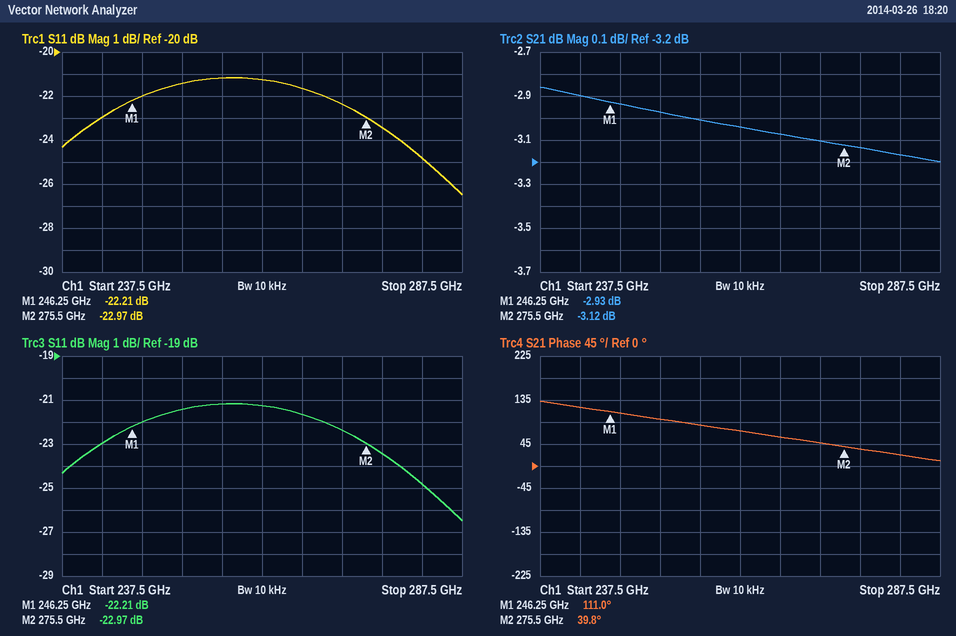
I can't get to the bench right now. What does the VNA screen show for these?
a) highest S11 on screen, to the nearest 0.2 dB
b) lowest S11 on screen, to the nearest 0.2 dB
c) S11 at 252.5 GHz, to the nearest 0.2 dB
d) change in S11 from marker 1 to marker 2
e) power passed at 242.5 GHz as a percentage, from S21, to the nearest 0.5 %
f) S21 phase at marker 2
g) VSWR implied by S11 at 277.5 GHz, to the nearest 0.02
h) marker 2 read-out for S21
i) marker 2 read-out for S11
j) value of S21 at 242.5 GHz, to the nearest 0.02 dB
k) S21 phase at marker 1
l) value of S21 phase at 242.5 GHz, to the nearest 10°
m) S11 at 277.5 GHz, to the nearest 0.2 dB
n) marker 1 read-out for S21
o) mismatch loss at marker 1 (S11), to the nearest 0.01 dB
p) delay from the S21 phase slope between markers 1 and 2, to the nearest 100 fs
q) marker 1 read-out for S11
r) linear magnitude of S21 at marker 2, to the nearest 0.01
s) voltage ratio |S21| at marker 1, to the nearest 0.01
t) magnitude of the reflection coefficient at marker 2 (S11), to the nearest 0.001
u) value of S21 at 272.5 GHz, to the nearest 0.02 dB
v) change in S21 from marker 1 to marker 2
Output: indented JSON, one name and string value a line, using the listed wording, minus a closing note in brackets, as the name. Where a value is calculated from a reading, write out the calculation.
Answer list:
{
  "highest S11 on screen, to the nearest 0.2 dB": "-21.2 dB",
  "lowest S11 on screen, to the nearest 0.2 dB": "-26.4 dB",
  "S11 at 252.5 GHz, to the nearest 0.2 dB": "-21.4 dB",
  "change in S11 from marker 1 to marker 2": "-22.97 − (-22.21) = -0.76 dB",
  "power passed at 242.5 GHz as a percentage, from S21, to the nearest 0.5 %": "10^(-2.9/10) ≈ 51.3 %, so 51.5 % to the nearest 0.5 %",
  "S21 phase at marker 2": "39.8°",
  "VSWR implied by S11 at 277.5 GHz, to the nearest 0.02": "|Γ| = 10^(-23.4/20) = 0.0676; VSWR = (1 + 0.0676)/(1 − 0.0676) ≈ 1.15, so 1.14 to the nearest 0.02",
  "marker 2 read-out for S21": "-3.12 dB",
  "marker 2 read-out for S11": "-22.97 dB",
  "value of S21 at 242.5 GHz, to the nearest 0.02 dB": "-2.90 dB",
  "S21 phase at marker 1": "111.0°",
  "value of S21 phase at 242.5 GHz, to the nearest 10°": "120°",
  "S11 at 277.5 GHz, to the nearest 0.2 dB": "-23.4 dB",
  "marker 1 read-out for S21": "-2.93 dB",
  "mismatch loss at marker 1 (S11), to the nearest 0.01 dB": "−10 log10(1 − 10^(-22.21/10)) ≈ 0.03 dB",
  "delay from the S21 phase slope between markers 1 and 2, to the nearest 100 fs": "−(39.8° − (111°))/(360° × 29.25 GHz) ≈ 6.8 ps",
  "marker 1 read-out for S11": "-22.21 dB",
  "linear magnitude of S21 at marker 2, to the nearest 0.01": "10^(-3.12/20) ≈ 0.70",
  "voltage ratio |S21| at marker 1, to the nearest 0.01": "10^(-2.93/20) ≈ 0.71",
  "magnitude of the reflection coefficient at marker 2 (S11), to the nearest 0.001": "10^(-22.97/20) ≈ 0.071",
  "value of S21 at 272.5 GHz, to the nearest 0.02 dB": "-3.10 dB",
  "change in S21 from marker 1 to marker 2": "-3.12 − (-2.93) = -0.19 dB"
}
